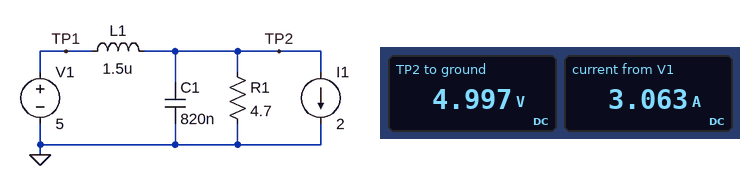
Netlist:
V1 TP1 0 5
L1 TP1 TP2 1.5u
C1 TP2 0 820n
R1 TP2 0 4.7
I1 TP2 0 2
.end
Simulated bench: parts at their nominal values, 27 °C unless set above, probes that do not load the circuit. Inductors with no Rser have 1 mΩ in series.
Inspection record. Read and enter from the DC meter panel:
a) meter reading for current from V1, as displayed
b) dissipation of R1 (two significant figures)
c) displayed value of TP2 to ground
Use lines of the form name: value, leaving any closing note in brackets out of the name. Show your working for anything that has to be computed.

meter reading for current from V1, as displayed: 3.063 A
dissipation of R1: (4.997 V)^2 / 4.7 Ω = 5.3 W
displayed value of TP2 to ground: 4.997 V
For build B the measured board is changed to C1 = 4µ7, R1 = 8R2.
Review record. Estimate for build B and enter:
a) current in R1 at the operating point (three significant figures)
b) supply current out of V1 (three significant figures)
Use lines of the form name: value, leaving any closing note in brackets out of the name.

current in R1 at the operating point: 609 mA
supply current out of V1: 2.61 A
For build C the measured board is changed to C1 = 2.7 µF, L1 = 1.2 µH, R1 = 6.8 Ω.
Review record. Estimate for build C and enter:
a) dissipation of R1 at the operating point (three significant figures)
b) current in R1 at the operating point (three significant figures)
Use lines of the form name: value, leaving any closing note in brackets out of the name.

dissipation of R1 at the operating point: 3.67 W
current in R1 at the operating point: 735 mA
